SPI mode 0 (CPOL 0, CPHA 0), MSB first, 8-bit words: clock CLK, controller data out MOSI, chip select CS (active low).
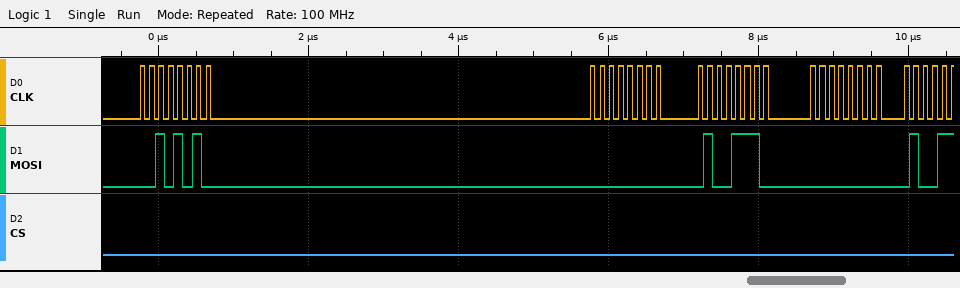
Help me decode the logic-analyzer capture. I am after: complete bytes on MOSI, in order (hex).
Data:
2A 00 4E 00
